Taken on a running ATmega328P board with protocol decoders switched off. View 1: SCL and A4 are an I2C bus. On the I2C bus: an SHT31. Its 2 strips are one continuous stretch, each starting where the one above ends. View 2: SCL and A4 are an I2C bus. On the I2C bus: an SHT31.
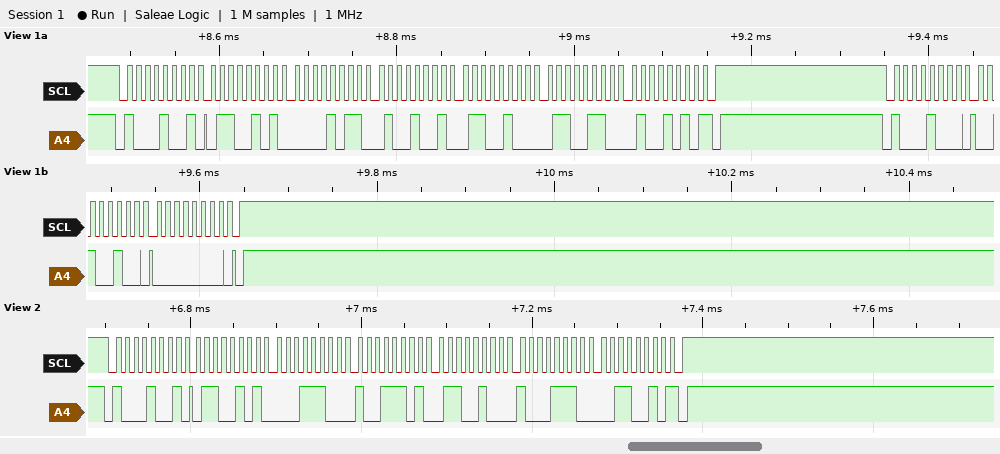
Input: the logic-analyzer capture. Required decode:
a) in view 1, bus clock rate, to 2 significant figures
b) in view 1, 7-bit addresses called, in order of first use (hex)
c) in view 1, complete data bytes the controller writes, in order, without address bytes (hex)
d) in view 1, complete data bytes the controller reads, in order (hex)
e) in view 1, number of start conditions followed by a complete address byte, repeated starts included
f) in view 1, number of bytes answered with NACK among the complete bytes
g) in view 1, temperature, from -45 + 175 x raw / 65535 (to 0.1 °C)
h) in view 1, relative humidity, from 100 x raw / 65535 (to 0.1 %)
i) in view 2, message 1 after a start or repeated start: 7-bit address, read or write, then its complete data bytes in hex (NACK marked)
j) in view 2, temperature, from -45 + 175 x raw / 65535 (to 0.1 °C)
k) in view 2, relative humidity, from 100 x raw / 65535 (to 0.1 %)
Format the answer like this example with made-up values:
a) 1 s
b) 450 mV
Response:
a) 100 kHz
b) 0x44
c) 24 00
d) 65 0B 49 64 66 4A
e) 2
f) 1
g) 24.1 °C
h) 39.2 %
i) 0x44 read: 65 1C 9D 64 8E 32 NACK
j) 24.1 °C
k) 39.3 %
